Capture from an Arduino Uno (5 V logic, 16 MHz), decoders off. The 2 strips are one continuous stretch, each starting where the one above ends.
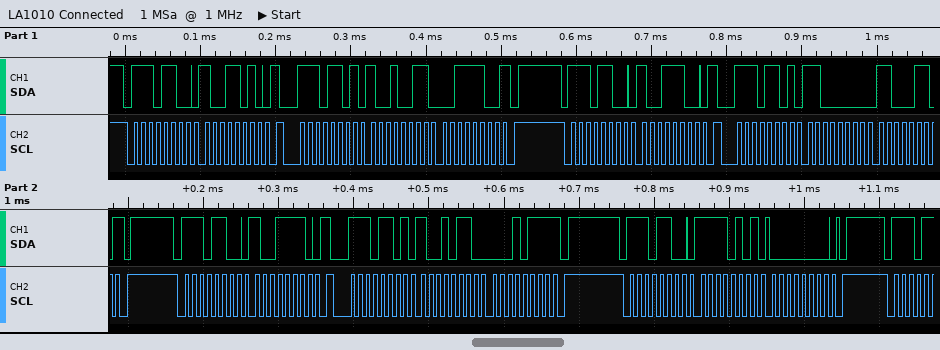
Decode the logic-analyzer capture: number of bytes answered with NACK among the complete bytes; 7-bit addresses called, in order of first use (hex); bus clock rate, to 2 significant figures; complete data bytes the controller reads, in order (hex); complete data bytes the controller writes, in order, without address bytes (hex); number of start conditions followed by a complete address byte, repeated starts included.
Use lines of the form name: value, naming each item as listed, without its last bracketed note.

number of bytes answered with NACK among the complete bytes: 3
7-bit addresses called, in order of first use: 0x76
bus clock rate, to 2 significant figures: 100 kHz
complete data bytes the controller reads, in order: 93 3C C0 C6 96 17
complete data bytes the controller writes, in order, without address bytes: 9A 9C 9E F5 00
number of start conditions followed by a complete address byte, repeated starts included: 7
